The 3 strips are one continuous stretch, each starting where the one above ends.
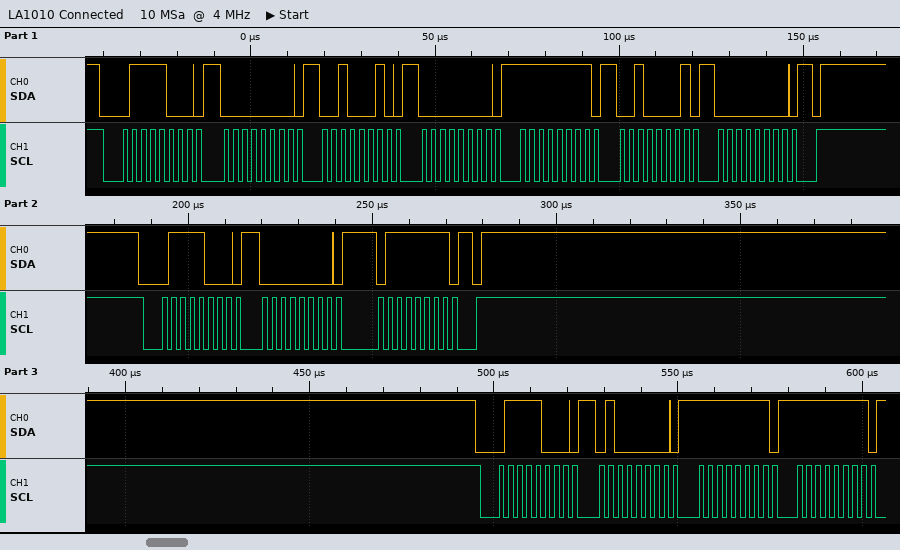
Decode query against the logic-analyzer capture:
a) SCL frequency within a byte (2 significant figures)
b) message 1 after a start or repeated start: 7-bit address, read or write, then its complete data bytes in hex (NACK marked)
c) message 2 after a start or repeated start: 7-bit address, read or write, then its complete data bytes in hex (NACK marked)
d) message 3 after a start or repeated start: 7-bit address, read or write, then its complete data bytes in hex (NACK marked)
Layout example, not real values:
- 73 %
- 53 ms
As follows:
- 400 kHz
- 0x3C write: 00 22 00 FF 21 00
- 0x3C write: 00 7F
- 0x3C write: 40 FF FF
